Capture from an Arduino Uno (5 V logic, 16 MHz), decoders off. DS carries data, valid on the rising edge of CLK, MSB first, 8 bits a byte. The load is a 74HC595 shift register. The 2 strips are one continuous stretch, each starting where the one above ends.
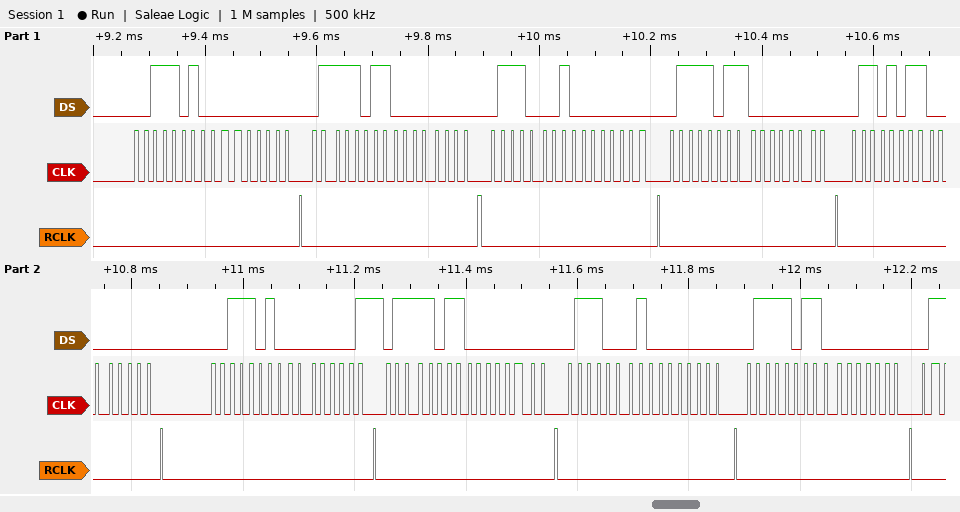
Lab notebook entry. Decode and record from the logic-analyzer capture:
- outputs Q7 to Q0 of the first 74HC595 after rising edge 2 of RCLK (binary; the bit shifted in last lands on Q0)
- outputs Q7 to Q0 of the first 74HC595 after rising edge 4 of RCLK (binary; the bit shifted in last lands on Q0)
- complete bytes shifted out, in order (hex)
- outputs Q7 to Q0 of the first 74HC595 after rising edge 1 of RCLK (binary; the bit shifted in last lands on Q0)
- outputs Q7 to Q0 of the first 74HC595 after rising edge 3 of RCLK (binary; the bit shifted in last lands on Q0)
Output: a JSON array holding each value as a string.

["00000000", "00000000", "0x3A 0x00 0x7B 0x00 0x71 0x00 0x7B 0x00 0x6B 0x00 0x3A 0x01 0x7B 0x00 0x71 0x00 0x7B 0x00", "00000000", "00000000"]
